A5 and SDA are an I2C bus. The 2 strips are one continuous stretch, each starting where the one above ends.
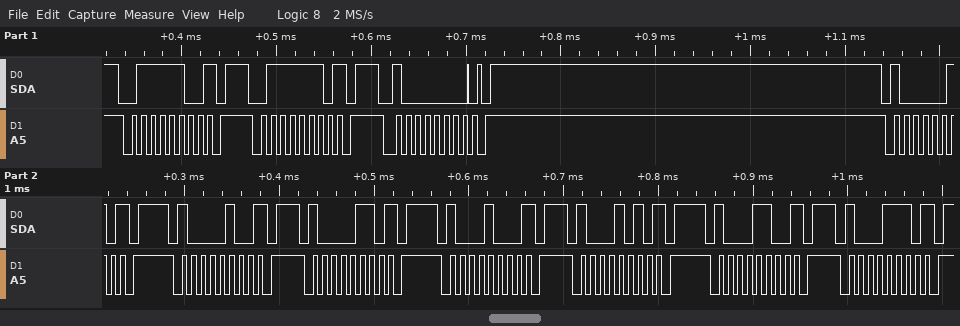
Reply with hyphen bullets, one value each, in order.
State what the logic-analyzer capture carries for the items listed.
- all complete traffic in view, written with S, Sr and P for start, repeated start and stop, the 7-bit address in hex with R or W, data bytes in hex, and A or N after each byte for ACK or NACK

- S 3EW N P S 3FW N P S 40W A P S 41W N P S 42W N P S 43W N P S 44W N P S 45W N P S 46W N P S 47W N P
